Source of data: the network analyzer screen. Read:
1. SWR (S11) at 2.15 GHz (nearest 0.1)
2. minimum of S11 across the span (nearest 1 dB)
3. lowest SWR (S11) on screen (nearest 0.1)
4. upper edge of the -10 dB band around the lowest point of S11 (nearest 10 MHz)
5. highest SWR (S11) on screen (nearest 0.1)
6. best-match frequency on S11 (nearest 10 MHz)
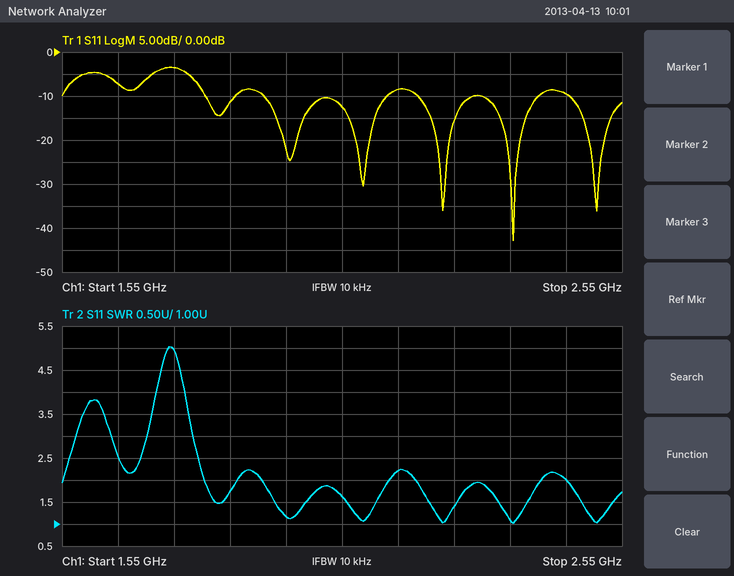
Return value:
2.2
-43 dB
1.0
2.40 GHz
5.0
2.36 GHz
